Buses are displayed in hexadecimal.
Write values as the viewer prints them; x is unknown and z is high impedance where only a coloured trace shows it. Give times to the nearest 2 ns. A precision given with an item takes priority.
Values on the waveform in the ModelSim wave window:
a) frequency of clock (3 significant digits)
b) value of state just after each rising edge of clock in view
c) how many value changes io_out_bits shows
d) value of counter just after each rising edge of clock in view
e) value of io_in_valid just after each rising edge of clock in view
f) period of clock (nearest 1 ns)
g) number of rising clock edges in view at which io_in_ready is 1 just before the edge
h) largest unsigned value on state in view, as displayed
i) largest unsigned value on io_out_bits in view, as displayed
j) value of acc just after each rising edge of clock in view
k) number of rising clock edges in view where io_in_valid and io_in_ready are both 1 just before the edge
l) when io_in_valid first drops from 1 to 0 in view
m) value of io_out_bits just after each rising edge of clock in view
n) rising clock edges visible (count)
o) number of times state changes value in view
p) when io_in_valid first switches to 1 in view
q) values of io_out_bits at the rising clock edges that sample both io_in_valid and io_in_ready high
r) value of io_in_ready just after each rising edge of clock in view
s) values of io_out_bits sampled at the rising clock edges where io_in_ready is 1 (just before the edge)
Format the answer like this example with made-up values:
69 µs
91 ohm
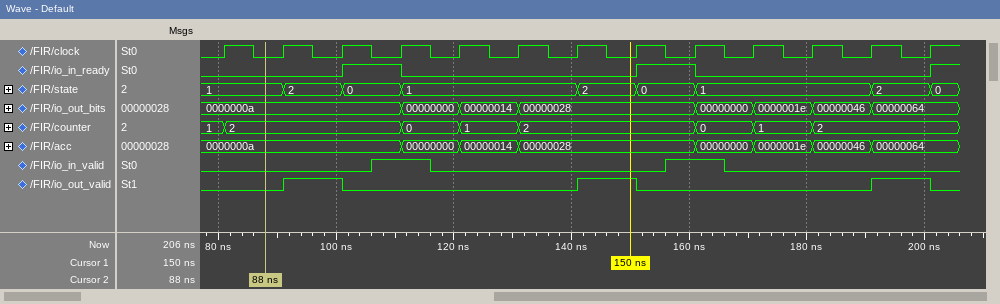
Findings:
100 MHz
1, 2, 0, 1, 1, 1, 2, 0, 1, 1, 1, 2, 0
7
2, 2, 2, 0, 1, 2, 2, 2, 0, 1, 2, 2, 2
0 0 0 1 0 0 0 0 1 0 0 0 0
10 ns
2
2
00000064
0000000a, 0000000a, 0000000a, 00000000, 00000014, 00000028, 00000028, 00000028, 00000000, 0000001e, 00000046, 00000064, 00000064
2
116 ns
0000000a, 0000000a, 0000000a, 00000000, 00000014, 00000028, 00000028, 00000028, 00000000, 0000001e, 00000046, 00000064, 00000064
13
8
106 ns
0000000a, 00000028
0 0 1 0 0 0 0 1 0 0 0 0 1
0000000a, 00000028
